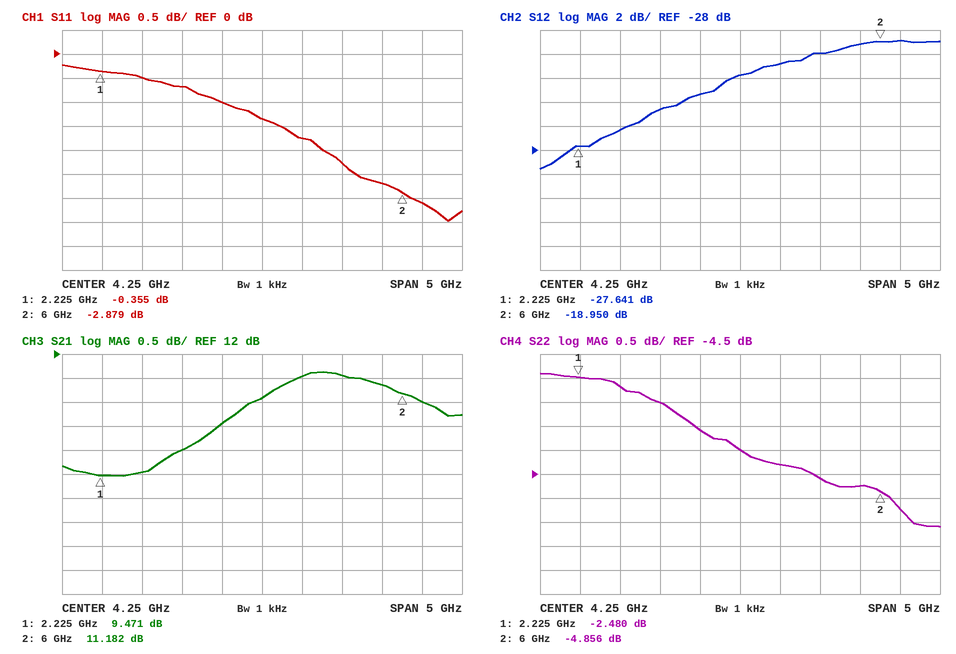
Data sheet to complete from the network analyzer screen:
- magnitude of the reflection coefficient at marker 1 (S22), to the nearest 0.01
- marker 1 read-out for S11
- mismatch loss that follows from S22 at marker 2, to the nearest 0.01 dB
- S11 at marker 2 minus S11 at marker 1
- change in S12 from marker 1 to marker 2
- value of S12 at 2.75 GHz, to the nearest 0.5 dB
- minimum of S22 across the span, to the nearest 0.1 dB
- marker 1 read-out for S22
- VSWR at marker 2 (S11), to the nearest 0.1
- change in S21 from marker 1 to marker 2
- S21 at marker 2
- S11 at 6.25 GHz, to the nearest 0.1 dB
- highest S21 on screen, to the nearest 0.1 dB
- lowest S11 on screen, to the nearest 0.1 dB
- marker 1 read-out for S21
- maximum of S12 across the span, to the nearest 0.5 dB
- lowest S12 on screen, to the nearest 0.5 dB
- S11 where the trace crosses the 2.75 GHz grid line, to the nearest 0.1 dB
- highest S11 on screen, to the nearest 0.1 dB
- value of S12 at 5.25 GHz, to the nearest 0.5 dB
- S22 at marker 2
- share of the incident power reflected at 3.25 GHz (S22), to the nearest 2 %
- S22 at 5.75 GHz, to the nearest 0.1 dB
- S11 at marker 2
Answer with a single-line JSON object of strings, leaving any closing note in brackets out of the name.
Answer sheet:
{"magnitude of the reflection coefficient at marker 1 (S22), to the nearest 0.01": "0.75", "marker 1 read-out for S11": "-0.355 dB", "mismatch loss that follows from S22 at marker 2, to the nearest 0.01 dB": "1.72 dB", "S11 at marker 2 minus S11 at marker 1": "-2.524 dB", "change in S12 from marker 1 to marker 2": "8.691 dB", "value of S12 at 2.75 GHz, to the nearest 0.5 dB": "-26.5 dB", "minimum of S22 across the span, to the nearest 0.1 dB": "-5.6 dB", "marker 1 read-out for S22": "-2.480 dB", "VSWR at marker 2 (S11), to the nearest 0.1": "6.1", "change in S21 from marker 1 to marker 2": "1.711 dB", "S21 at marker 2": "11.182 dB", "S11 at 6.25 GHz, to the nearest 0.1 dB": "-3.1 dB", "highest S21 on screen, to the nearest 0.1 dB": "11.6 dB", "lowest S11 on screen, to the nearest 0.1 dB": "-3.5 dB", "marker 1 read-out for S21": "9.471 dB", "maximum of S12 across the span, to the nearest 0.5 dB": "-19.0 dB", "lowest S12 on screen, to the nearest 0.5 dB": "-29.5 dB", "S11 where the trace crosses the 2.75 GHz grid line, to the nearest 0.1 dB": "-0.5 dB", "highest S11 on screen, to the nearest 0.1 dB": "-0.2 dB", "value of S12 at 5.25 GHz, to the nearest 0.5 dB": "-20.0 dB", "S22 at marker 2": "-4.856 dB", "share of the incident power reflected at 3.25 GHz (S22), to the nearest 2 %": "50 %", "S22 at 5.75 GHz, to the nearest 0.1 dB": "-4.7 dB", "S11 at marker 2": "-2.879 dB"}
